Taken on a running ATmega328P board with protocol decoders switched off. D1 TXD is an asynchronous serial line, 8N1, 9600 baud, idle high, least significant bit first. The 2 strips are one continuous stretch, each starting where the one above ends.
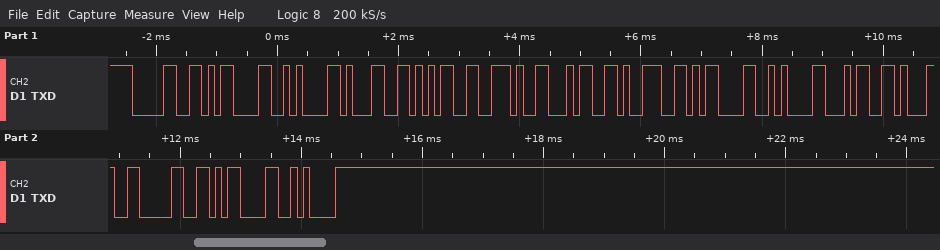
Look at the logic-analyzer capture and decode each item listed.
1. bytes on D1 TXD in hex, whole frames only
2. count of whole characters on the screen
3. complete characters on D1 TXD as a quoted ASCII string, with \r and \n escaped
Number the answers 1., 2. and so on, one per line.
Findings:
1. 30 0D 0A 31 35 2E 34 39 0D 0A 34 31 30 0D 0A
2. 15
3. "0\r\n15.49\r\n410\r\n"
